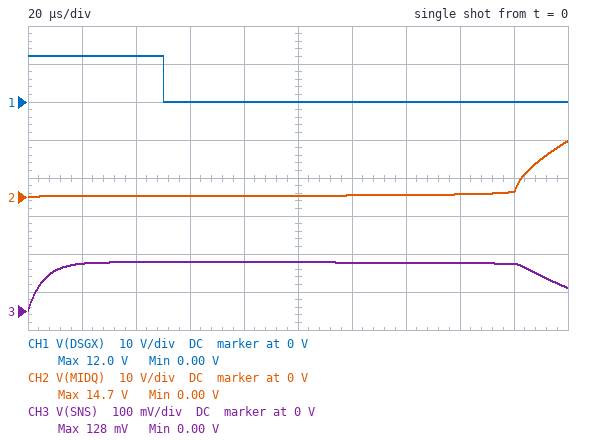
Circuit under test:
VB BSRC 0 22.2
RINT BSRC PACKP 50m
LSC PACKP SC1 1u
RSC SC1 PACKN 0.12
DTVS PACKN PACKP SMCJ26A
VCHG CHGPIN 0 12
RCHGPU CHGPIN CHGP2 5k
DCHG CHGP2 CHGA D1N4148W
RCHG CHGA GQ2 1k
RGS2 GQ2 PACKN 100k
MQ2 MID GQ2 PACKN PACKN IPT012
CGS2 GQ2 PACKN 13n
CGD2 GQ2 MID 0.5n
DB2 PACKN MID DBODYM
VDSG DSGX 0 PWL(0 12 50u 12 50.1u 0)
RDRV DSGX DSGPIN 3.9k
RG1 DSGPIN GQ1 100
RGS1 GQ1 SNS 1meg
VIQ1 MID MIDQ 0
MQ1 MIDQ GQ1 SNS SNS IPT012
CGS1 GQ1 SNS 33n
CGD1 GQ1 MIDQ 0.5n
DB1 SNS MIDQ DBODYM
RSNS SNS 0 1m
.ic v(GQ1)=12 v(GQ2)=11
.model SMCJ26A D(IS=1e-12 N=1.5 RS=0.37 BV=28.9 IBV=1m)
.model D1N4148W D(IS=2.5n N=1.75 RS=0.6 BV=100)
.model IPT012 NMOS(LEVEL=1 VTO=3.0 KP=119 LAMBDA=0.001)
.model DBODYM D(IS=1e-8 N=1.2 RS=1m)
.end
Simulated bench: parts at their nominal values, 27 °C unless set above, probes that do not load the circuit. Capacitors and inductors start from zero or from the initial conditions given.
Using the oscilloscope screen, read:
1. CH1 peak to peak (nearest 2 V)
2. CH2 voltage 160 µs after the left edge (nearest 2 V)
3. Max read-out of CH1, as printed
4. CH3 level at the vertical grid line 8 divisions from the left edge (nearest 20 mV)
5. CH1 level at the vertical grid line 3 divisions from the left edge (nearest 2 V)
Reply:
12 V
0 V
12.0 V
120 mV
0 V
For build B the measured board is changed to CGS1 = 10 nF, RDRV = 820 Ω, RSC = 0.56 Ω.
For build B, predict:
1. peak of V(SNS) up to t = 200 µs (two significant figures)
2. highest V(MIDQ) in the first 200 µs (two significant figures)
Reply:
36 mV
25 V
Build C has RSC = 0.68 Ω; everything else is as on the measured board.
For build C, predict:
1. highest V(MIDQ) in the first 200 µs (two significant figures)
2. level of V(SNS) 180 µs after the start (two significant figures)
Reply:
390 mV
30 mV
